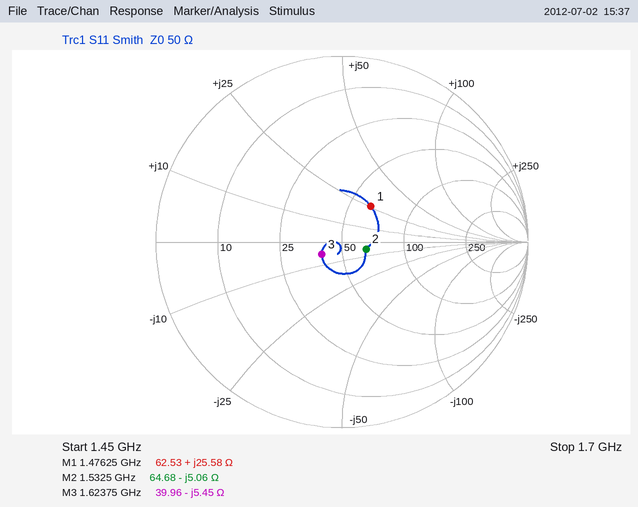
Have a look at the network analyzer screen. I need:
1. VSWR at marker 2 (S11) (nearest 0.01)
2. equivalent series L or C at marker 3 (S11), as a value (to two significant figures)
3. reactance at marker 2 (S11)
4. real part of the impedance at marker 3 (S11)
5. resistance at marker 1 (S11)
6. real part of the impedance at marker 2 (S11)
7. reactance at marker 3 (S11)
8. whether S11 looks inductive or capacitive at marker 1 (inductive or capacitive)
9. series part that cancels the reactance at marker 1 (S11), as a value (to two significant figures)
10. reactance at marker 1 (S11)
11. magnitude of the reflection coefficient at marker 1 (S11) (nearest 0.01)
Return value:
1.31
18 pF
-5.06 Ω
39.96 Ω
62.53 Ω
64.68 Ω
-5.45 Ω
inductive
4.2 pF
+25.58 Ω
0.25
